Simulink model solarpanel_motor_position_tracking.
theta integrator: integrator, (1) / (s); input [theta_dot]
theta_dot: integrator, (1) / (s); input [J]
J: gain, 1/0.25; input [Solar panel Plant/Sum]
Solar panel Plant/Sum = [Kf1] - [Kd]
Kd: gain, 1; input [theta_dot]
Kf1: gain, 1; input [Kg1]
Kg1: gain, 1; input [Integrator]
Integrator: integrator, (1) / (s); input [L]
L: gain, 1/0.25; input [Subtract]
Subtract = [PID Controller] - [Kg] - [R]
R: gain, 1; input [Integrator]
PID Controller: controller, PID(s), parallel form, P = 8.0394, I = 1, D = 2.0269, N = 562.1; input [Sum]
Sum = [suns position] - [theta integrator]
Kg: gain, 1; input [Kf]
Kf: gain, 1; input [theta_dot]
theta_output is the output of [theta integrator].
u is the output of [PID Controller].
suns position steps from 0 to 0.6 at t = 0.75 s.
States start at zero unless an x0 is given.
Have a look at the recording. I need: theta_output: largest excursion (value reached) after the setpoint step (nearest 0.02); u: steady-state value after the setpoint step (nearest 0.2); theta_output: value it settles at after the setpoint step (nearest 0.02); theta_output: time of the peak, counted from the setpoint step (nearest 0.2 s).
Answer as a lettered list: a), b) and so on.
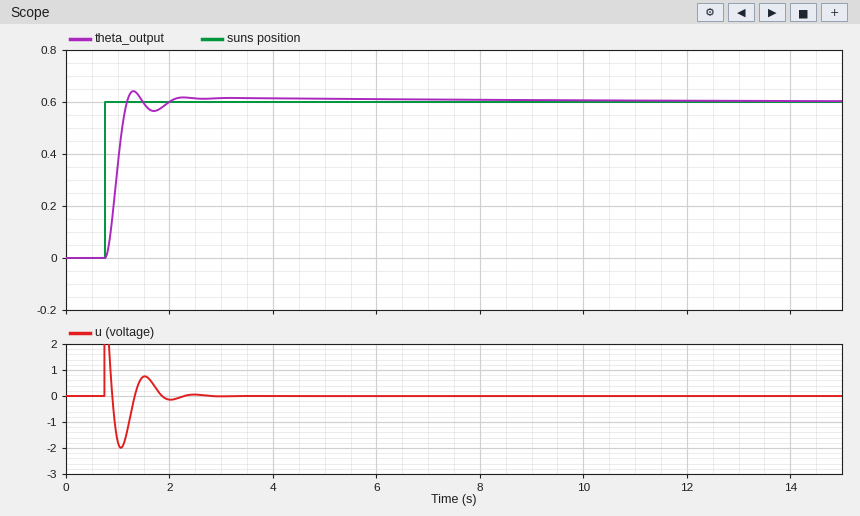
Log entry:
a) 0.64
b) 0.0
c) 0.60
d) 0.6 s
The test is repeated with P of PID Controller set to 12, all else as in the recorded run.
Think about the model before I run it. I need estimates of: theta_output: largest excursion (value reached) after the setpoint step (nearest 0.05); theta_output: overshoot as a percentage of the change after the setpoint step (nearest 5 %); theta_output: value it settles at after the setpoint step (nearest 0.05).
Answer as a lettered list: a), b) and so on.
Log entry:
a) 0.75
b) 25 %
c) 0.60
